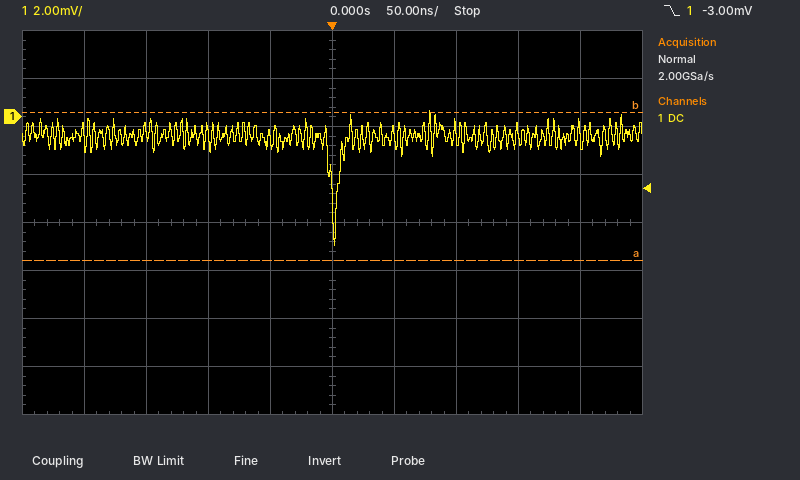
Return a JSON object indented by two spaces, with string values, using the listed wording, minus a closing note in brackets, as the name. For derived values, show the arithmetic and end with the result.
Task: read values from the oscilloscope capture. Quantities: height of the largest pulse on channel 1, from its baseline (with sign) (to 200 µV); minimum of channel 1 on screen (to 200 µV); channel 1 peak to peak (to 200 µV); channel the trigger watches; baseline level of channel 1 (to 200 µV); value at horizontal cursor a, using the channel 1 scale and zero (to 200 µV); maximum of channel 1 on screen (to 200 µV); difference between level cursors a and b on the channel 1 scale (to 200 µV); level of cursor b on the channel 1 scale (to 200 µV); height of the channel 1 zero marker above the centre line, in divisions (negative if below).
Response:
{
  "height of the largest pulse on channel 1, from its baseline (with sign)": "-5.4 mV − (-800 µV) = -4.6 mV",
  "minimum of channel 1 on screen": "-5.4 mV",
  "channel 1 peak to peak": "200 µV − (-5.4 mV) = 5.6 mV",
  "channel the trigger watches": "channel 1",
  "baseline level of channel 1": "-800 µV",
  "value at horizontal cursor a, using the channel 1 scale and zero": "-6.0 mV",
  "maximum of channel 1 on screen": "200 µV",
  "difference between level cursors a and b on the channel 1 scale": "6.2 mV",
  "level of cursor b on the channel 1 scale": "200 µV",
  "height of the channel 1 zero marker above the centre line, in divisions": "+2.2 div"
}
